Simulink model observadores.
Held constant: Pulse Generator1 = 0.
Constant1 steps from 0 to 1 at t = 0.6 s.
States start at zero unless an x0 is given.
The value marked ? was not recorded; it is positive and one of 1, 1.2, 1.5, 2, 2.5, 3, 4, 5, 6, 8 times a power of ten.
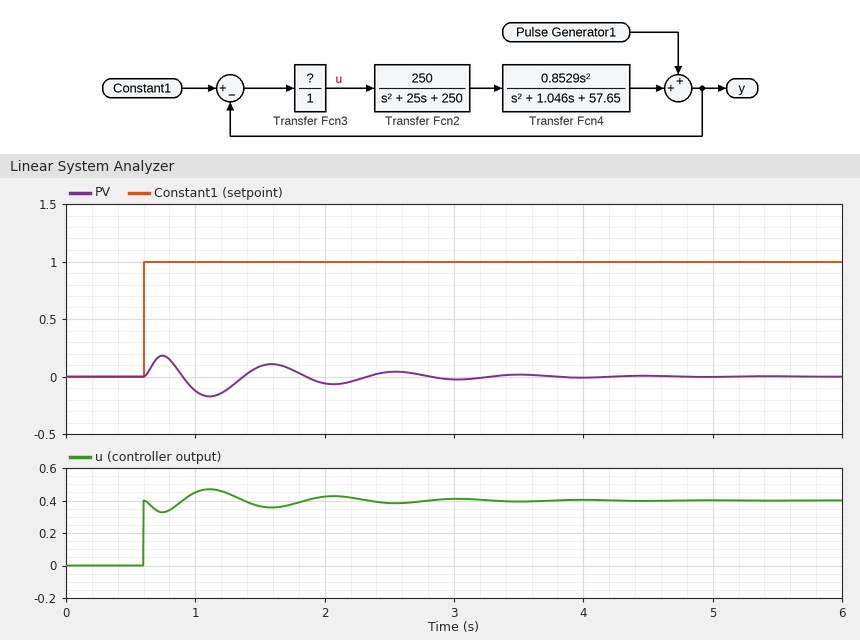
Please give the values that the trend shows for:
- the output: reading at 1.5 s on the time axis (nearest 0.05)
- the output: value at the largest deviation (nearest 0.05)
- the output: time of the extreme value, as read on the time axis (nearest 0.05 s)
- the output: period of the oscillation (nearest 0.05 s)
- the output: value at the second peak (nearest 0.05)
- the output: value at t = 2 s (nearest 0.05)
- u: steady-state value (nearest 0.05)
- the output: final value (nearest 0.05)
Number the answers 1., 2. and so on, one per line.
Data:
1. 0.10
2. 0.20
3. 0.75 s
4. 0.85 s
5. 0.10
6. -0.05
7. 0.40
8. 0.00
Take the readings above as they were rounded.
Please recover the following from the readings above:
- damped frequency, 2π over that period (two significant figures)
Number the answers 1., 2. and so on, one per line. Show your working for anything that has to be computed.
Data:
1. 2π / 0.85 = 7.4 rad/s
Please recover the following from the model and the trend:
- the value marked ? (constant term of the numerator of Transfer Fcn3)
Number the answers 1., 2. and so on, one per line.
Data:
1. 0.4
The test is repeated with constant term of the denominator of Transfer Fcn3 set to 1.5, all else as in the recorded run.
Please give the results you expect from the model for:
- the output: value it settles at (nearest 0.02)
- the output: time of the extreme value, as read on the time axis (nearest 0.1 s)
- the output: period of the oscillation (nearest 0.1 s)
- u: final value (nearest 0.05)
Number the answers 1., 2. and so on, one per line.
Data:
1. 0.00
2. 1.1 s
3. 0.9 s
4. 0.25
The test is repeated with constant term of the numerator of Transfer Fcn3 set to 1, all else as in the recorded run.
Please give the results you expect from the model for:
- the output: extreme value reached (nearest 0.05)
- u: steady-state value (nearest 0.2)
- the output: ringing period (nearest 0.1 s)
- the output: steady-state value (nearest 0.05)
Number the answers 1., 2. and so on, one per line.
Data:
1. 0.40
2. 1.0
3. 1.0 s
4. 0.00
